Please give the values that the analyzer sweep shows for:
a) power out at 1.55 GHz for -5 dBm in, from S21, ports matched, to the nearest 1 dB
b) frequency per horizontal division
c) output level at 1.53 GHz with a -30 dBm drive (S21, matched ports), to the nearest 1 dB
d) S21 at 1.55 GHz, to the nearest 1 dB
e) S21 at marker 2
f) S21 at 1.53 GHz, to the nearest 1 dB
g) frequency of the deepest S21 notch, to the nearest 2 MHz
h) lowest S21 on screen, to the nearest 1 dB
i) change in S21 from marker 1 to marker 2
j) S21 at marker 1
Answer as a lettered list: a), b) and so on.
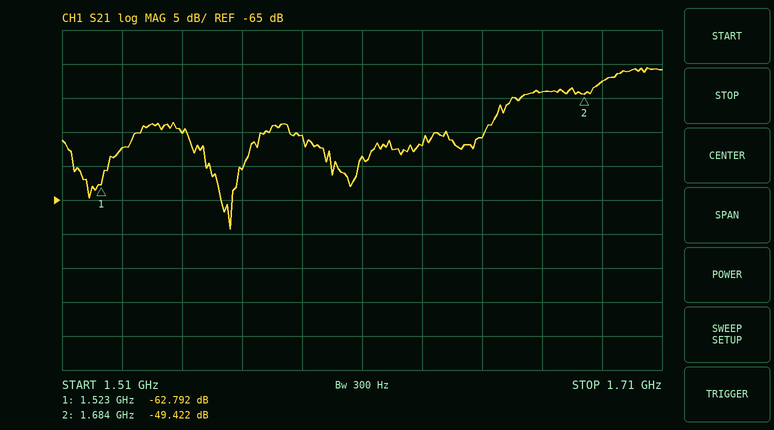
a) -60 dBm
b) 20 MHz
c) -87 dBm
d) -55 dB
e) -49.422 dB
f) -57 dB
g) 1.566 GHz
h) -69 dB
i) 13.370 dB
j) -62.792 dB
